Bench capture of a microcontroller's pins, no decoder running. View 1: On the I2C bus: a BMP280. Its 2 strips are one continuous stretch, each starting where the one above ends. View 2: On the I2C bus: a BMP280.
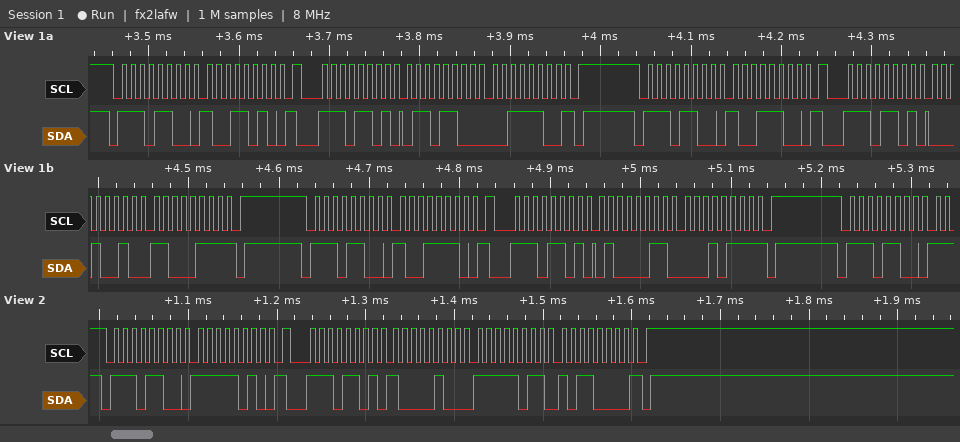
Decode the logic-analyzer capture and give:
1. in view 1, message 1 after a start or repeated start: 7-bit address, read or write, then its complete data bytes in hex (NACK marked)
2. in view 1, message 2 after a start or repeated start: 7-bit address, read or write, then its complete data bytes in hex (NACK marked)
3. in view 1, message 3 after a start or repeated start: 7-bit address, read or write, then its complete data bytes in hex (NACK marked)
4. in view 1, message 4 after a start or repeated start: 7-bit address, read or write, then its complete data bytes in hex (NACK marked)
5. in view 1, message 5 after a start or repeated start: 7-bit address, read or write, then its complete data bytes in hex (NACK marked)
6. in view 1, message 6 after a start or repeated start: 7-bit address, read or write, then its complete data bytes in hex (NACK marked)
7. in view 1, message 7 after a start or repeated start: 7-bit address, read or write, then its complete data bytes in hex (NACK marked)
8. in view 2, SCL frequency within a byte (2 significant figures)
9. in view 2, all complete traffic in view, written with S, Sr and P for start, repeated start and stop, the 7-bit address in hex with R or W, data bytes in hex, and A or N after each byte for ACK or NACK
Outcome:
0x76 write: 9A
0x76 read: 6C 3C NACK
0x76 write: 9C
0x76 read: 12 C7 NACK
0x76 write: 9E
0x76 read: 43 17 NACK
0x76 write
100 kHz
S 76W A FA A Sr 76R A 84 A FB A B0 N P
